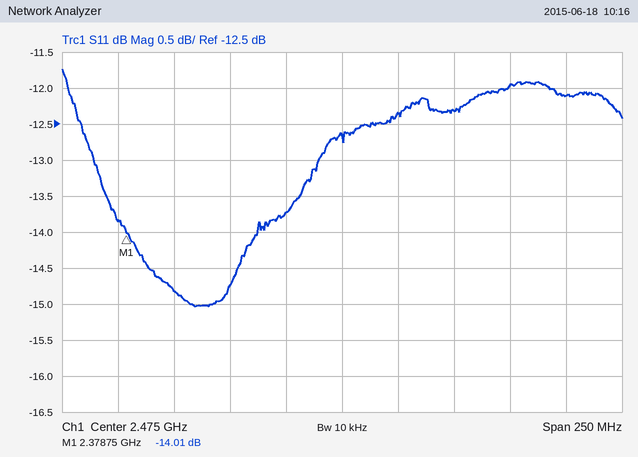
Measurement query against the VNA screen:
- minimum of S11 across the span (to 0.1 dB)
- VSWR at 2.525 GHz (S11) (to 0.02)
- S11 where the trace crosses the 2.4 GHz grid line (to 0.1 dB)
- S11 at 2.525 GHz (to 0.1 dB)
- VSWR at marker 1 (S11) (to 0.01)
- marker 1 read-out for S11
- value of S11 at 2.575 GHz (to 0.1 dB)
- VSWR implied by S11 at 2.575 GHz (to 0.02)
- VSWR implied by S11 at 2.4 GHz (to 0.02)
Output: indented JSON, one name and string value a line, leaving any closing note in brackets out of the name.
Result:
{
  "minimum of S11 across the span": "-15.0 dB",
  "VSWR at 2.525 GHz (S11)": "1.64",
  "S11 where the trace crosses the 2.4 GHz grid line": "-14.8 dB",
  "S11 at 2.525 GHz": "-12.3 dB",
  "VSWR at marker 1 (S11)": "1.50",
  "marker 1 read-out for S11": "-14.01 dB",
  "value of S11 at 2.575 GHz": "-12.1 dB",
  "VSWR implied by S11 at 2.575 GHz": "1.66",
  "VSWR implied by S11 at 2.4 GHz": "1.44"
}
